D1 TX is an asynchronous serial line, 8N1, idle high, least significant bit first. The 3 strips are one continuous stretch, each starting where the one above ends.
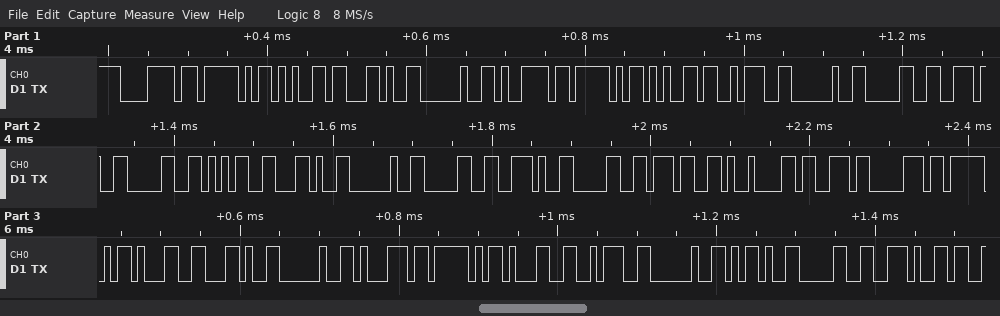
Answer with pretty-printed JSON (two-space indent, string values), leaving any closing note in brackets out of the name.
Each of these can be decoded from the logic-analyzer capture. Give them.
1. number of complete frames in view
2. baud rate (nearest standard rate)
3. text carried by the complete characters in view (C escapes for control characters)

{
  "number of complete frames in view": "35",
  "baud rate": "115200 baud",
  "text carried by the complete characters in view": "\"x_e, y_e: 0.05, 0.07\\tsp_1, q_1: -0.\""
}
